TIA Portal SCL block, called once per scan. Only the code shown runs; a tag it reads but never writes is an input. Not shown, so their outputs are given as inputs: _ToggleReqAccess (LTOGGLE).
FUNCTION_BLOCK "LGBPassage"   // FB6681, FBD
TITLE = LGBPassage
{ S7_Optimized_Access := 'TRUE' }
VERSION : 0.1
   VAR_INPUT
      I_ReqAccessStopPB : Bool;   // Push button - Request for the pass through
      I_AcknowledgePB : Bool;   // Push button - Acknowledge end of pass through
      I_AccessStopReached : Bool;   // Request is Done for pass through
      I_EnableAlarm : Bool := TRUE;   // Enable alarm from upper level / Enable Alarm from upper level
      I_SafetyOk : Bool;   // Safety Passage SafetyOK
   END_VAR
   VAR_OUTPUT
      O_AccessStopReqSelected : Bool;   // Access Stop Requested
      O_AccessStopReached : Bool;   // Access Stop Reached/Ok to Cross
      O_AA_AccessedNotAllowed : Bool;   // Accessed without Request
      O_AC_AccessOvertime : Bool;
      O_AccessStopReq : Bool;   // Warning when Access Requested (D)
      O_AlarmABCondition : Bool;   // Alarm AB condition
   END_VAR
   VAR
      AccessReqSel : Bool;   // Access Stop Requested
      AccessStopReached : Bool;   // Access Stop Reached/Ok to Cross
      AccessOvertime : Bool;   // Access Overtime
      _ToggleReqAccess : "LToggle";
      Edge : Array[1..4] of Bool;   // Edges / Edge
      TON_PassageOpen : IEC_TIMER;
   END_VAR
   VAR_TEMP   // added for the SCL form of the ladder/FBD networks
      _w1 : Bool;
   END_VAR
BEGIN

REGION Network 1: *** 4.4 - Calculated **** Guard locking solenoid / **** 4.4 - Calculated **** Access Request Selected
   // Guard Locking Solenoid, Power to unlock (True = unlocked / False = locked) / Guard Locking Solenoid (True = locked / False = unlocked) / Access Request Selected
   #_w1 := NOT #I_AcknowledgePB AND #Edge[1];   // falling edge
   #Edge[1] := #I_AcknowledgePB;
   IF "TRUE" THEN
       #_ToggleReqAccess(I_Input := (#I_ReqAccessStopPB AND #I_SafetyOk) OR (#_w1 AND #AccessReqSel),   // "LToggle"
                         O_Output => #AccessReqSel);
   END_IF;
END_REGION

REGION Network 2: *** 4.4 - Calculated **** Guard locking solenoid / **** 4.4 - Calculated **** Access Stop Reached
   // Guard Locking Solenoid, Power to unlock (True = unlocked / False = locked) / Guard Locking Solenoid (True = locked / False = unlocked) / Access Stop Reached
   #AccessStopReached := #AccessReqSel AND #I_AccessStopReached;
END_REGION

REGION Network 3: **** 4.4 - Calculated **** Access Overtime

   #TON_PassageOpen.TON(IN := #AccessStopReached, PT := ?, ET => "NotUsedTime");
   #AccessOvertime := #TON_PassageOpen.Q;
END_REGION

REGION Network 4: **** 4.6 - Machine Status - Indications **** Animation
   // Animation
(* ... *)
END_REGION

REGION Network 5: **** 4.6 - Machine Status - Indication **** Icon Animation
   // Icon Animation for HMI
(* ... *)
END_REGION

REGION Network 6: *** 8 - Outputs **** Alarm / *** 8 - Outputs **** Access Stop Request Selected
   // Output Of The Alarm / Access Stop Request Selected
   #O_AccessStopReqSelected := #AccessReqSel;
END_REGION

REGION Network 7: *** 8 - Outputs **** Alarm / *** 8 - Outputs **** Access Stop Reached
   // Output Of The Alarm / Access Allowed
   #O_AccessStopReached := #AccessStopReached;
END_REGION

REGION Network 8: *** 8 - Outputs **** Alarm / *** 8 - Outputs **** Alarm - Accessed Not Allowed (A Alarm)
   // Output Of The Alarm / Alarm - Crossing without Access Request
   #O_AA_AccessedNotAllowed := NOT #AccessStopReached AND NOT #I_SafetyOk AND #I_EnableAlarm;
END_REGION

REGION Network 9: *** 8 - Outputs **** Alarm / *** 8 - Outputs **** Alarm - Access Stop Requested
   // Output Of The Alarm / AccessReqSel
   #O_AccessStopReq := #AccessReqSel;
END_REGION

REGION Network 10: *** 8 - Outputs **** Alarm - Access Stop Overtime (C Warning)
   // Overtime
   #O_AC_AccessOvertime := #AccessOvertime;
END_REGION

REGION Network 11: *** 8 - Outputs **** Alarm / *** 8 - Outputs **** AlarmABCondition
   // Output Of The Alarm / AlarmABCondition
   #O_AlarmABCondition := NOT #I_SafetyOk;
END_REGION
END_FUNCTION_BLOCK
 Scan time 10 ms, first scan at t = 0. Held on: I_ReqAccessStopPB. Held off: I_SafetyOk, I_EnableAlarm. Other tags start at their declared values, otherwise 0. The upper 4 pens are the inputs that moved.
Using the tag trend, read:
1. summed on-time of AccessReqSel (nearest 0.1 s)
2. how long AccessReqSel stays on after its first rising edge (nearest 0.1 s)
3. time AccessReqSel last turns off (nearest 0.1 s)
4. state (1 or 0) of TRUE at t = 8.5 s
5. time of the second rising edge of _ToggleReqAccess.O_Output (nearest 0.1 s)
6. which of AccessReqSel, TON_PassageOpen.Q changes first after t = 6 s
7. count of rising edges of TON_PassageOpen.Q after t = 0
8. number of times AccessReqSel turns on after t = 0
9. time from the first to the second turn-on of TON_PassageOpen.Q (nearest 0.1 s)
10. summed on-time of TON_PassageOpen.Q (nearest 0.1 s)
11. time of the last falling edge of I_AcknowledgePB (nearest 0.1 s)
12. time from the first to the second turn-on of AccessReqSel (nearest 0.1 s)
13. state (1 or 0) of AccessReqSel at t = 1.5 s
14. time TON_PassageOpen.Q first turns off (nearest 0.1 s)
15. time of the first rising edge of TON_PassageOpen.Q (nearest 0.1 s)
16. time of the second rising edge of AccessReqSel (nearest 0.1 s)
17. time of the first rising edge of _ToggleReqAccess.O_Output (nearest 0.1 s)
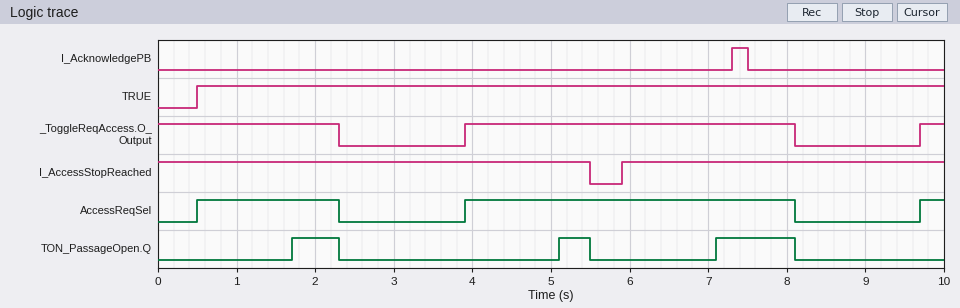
6.3 s
1.8 s
8.1 s
1
9.7 s
TON_PassageOpen.Q
3
3
3.4 s
2.0 s
7.5 s
3.4 s
1
2.3 s
1.7 s
3.9 s
3.9 s
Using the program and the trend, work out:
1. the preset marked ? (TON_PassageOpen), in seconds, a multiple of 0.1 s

1.2 s
